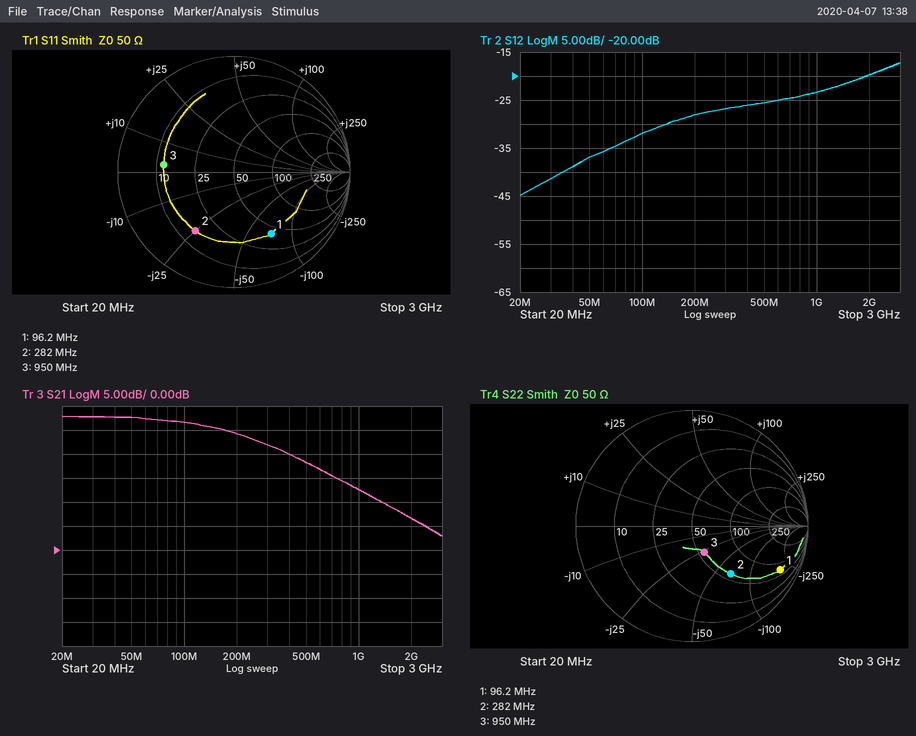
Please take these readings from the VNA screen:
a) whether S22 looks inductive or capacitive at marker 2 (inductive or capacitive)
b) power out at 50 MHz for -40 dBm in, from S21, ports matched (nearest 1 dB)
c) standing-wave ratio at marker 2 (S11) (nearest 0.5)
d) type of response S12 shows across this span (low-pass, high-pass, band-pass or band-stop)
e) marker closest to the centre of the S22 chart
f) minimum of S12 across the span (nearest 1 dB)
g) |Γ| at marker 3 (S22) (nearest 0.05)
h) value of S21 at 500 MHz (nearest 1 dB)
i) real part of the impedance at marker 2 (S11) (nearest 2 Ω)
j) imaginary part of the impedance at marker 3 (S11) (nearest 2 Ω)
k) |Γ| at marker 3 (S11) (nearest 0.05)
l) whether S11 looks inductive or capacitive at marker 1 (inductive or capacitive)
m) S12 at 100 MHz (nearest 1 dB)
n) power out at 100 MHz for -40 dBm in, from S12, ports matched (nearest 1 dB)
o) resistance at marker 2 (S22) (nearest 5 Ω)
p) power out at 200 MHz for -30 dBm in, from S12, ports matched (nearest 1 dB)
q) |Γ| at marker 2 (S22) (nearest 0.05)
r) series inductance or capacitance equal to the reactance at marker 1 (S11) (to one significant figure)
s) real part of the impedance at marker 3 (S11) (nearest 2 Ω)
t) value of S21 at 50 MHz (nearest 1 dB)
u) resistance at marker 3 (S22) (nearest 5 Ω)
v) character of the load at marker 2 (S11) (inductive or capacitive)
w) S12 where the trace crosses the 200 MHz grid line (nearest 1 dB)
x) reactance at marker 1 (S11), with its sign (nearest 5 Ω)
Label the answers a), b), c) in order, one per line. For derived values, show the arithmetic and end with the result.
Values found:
a) capacitive
b) -40 dBm + (28 dB) = -12 dBm
c) 4.0
d) high-pass
e) marker 3
f) -45 dB
g) 0.25
h) 18 dB
i) 16 Ω
j) +2 Ω
k) 0.60
l) capacitive
m) -32 dB
n) -40 dBm + (-32 dB) = -72 dBm
o) 60 Ω
p) -30 dBm + (-28 dB) = -58 dBm
q) 0.55
r) C = 1/(2π × 96.2 MHz × 70 Ω) ≈ 23.6 pF, so 20 pF to one significant figure
s) 12 Ω
t) 28 dB
u) 55 Ω
v) capacitive
w) -28 dB
x) -70 Ω
